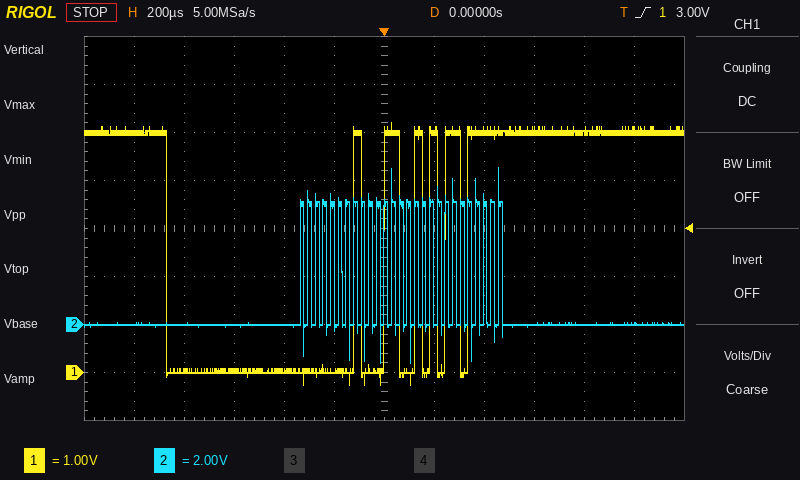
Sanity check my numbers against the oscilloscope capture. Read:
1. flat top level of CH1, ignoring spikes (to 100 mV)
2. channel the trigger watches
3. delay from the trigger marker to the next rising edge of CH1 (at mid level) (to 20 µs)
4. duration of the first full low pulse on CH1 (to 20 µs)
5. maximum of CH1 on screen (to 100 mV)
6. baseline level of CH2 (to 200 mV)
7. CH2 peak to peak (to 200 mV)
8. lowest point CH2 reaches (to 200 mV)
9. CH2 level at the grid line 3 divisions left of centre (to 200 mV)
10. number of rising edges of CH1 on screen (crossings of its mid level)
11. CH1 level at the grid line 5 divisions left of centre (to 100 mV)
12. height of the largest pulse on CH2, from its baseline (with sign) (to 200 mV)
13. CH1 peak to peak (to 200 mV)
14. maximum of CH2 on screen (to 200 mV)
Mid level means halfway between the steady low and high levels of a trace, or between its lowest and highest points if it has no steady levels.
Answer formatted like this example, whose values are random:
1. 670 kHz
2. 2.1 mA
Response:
1. 5.0 V
2. CH1
3. 120 µs
4. 740 µs
5. 5.2 V
6. 0.0 V
7. 8.2 V
8. -1.6 V
9. 0.0 V
10. 6
11. 5.0 V
12. +6.6 V
13. 5.4 V
14. 6.6 V
